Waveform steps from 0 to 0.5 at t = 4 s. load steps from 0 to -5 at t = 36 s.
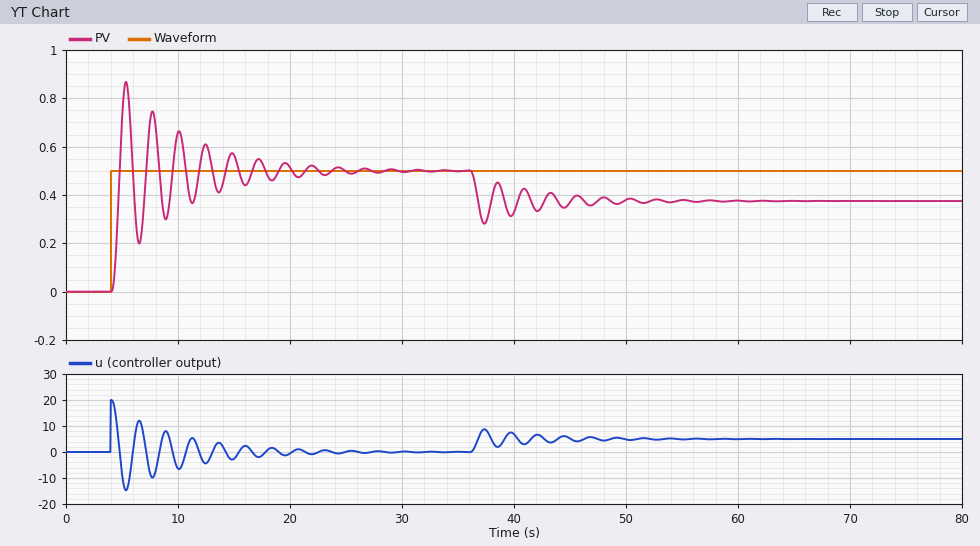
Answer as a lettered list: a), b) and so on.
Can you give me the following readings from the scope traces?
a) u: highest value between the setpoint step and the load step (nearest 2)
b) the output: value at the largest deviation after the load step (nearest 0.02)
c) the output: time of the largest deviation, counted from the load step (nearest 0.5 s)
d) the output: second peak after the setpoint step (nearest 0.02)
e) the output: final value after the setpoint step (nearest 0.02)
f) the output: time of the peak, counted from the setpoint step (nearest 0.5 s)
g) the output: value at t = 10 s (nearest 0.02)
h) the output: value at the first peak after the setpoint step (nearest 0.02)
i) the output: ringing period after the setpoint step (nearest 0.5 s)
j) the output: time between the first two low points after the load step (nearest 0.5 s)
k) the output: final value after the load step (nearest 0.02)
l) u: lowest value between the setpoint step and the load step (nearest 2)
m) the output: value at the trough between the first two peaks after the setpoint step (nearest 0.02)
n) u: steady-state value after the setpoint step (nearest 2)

a) 20
b) 0.28
c) 1.5 s
d) 0.74
e) 0.50
f) 1.5 s
g) 0.66
h) 0.86
i) 2.5 s
j) 2.5 s
k) 0.38
l) -14
m) 0.20
n) 0
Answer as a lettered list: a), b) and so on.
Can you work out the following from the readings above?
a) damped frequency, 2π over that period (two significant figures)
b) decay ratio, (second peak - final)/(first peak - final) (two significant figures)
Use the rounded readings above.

a) 2.5 rad/s
b) 0.67
